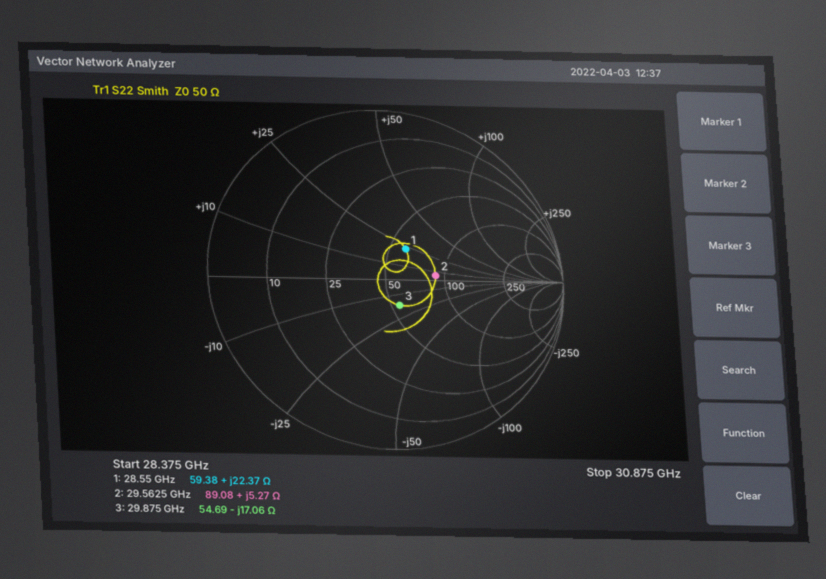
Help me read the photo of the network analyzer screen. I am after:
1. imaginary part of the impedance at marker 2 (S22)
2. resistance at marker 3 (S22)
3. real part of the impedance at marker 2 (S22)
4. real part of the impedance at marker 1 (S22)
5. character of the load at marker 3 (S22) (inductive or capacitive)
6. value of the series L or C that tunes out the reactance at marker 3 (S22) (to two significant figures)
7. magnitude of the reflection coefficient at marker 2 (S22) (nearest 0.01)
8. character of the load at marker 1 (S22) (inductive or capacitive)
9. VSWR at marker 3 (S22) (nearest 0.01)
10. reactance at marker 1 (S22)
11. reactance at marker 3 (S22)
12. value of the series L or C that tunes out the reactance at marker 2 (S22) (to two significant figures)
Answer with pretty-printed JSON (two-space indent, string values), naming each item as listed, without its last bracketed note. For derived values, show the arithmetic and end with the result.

{
  "imaginary part of the impedance at marker 2": "+5.27 Ω",
  "resistance at marker 3": "54.69 Ω",
  "real part of the impedance at marker 2": "89.08 Ω",
  "real part of the impedance at marker 1": "59.38 Ω",
  "character of the load at marker 3 (S22)": "capacitive",
  "value of the series L or C that tunes out the reactance at marker 3 (S22)": "L = 17.06 Ω/(2π × 29.875 GHz) ≈ 91 pH",
  "magnitude of the reflection coefficient at marker 2 (S22)": "0.28",
  "character of the load at marker 1 (S22)": "inductive",
  "VSWR at marker 3 (S22)": "1.40",
  "reactance at marker 1": "+22.37 Ω",
  "reactance at marker 3": "-17.06 Ω",
  "value of the series L or C that tunes out the reactance at marker 2 (S22)": "C = 1/(2π × 29.5625 GHz × 5.27 Ω) ≈ 1.0 pF"
}
